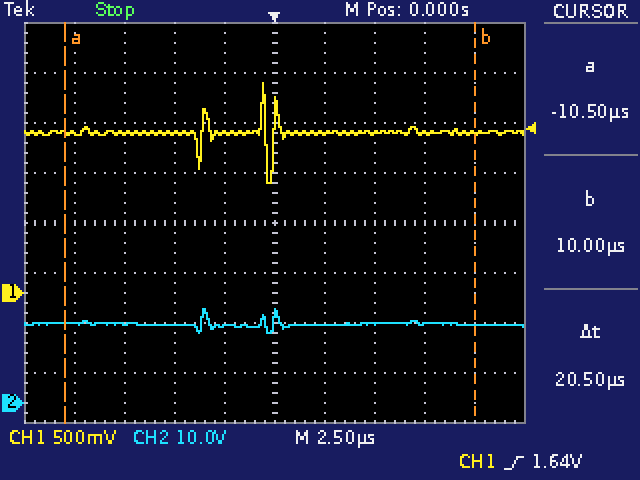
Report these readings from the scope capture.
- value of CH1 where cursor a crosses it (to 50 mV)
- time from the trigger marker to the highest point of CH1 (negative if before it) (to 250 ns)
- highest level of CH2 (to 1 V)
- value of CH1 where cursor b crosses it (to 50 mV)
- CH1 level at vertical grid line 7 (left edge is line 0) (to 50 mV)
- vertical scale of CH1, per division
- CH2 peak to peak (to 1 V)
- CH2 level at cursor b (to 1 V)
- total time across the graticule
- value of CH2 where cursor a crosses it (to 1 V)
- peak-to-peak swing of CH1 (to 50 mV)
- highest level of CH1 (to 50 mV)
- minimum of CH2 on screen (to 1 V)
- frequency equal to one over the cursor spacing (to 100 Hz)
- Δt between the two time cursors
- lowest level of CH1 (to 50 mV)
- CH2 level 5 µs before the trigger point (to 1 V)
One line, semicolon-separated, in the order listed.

1.60 V; -500 ns; 19 V; 1.60 V; 1.60 V; 500 mV; 5 V; 16 V; 25 µs; 16 V; 1.00 V; 2.10 V; 14 V; 48.8 kHz; 20.5 µs; 1.10 V; 16 V
